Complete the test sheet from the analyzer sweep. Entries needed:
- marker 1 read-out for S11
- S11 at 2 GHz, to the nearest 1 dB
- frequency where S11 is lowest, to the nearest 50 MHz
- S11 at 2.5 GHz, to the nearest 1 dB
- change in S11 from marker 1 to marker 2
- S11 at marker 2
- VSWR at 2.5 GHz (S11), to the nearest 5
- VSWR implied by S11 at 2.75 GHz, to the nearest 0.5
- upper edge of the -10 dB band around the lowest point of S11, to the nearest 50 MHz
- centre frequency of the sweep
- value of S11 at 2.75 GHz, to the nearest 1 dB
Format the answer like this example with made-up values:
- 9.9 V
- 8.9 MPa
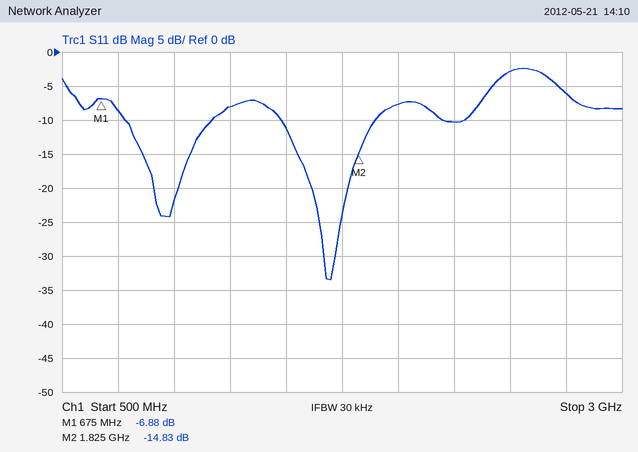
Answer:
- -6.88 dB
- -8 dB
- 1.70 GHz
- -3 dB
- -7.95 dB
- -14.83 dB
- 5
- 3.0
- 1.90 GHz
- 1.75 GHz
- -6 dB
